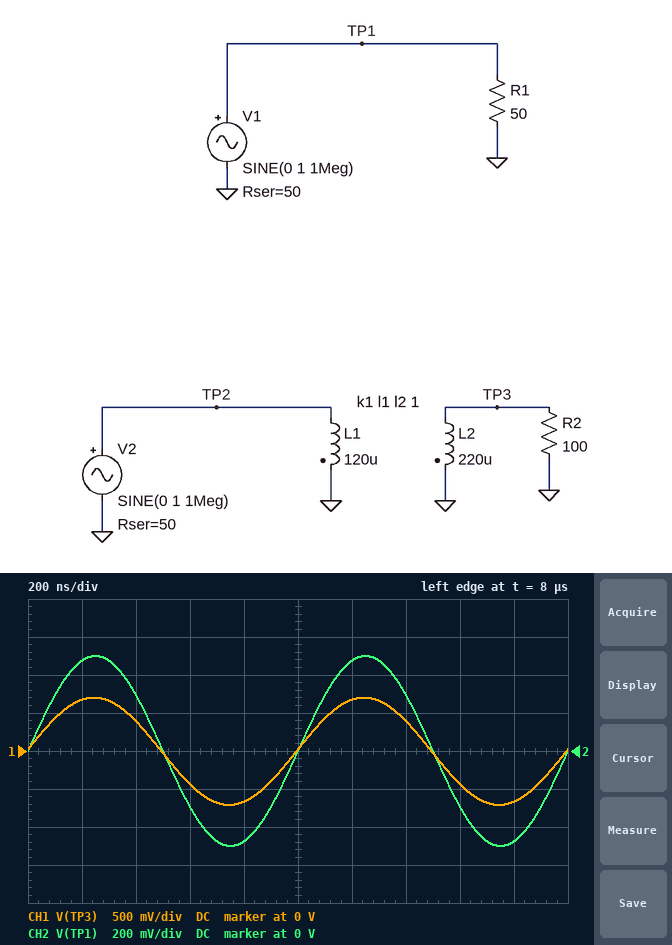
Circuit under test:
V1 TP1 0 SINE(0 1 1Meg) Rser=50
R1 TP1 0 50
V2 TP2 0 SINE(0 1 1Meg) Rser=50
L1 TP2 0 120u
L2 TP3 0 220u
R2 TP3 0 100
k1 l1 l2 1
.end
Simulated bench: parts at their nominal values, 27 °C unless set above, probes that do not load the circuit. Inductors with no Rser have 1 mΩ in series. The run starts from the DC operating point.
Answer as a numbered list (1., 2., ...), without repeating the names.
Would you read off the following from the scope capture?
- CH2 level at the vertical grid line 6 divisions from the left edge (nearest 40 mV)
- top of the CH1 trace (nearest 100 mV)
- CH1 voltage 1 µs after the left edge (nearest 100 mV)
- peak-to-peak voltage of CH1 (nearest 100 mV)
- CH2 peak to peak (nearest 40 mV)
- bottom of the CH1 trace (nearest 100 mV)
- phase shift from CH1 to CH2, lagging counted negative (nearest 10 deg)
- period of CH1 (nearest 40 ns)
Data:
1. 480 mV
2. 700 mV
3. 0 V
4. 1.4 V
5. 1.00 V
6. -700 mV
7. 0 deg
8. 1.00 µs
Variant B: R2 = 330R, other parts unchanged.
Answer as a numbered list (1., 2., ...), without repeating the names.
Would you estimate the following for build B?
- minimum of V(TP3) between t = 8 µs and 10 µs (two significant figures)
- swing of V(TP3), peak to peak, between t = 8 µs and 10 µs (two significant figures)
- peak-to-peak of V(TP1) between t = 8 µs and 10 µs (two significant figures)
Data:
1. -1.1 V
2. 2.1 V
3. 1.0 V
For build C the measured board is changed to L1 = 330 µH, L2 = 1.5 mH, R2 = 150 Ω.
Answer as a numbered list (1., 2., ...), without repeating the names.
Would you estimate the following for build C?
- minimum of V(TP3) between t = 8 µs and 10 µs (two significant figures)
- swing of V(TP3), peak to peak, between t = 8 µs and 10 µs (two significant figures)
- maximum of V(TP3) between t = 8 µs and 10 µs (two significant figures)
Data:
1. -850 mV
2. 1.7 V
3. 840 mV
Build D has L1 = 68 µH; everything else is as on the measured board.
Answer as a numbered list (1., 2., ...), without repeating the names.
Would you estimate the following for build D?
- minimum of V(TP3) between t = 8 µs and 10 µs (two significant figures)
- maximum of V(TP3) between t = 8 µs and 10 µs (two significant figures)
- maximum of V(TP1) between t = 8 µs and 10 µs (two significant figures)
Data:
1. -690 mV
2. 680 mV
3. 500 mV
